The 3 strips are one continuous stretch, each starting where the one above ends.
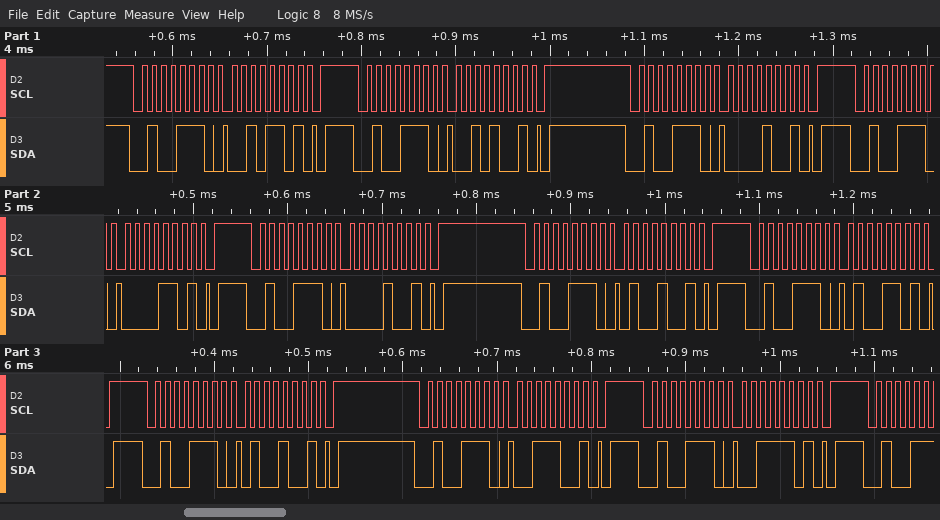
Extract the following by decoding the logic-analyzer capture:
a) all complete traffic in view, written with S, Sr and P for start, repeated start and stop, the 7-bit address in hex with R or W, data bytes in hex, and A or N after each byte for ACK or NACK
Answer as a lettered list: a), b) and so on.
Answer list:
a) S 27W A 2D A P S 27W A 29 A P S 27W A 09 A P S 27W A 0D A P S 27W A 09 A P S 27W A 49 A P S 27W A 4D A P S 27W A 49 A P S 27W A 39 A P S 27W A 3D A P
